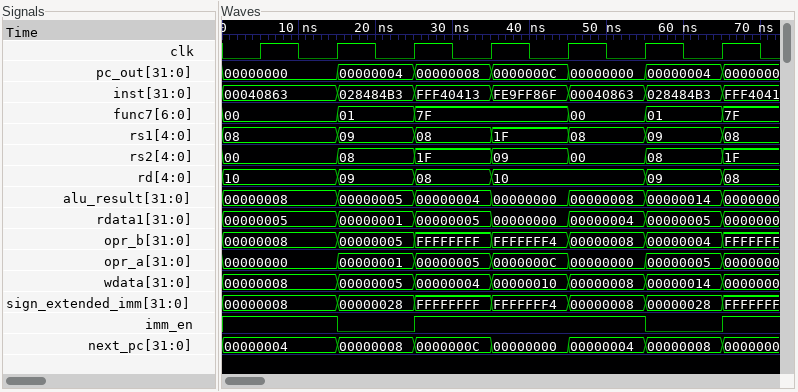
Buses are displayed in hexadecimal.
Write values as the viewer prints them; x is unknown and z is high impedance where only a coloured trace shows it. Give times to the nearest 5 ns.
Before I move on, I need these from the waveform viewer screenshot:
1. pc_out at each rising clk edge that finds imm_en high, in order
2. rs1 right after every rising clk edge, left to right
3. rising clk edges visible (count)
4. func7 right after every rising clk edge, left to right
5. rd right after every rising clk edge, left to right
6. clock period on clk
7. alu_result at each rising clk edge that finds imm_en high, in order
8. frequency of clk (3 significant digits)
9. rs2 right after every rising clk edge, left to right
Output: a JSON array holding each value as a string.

["00000000, 00000000, 00000008, 0000000C, 00000000", "08, 09, 08, 1F, 08, 09, 08", "7", "00, 01, 7F, 7F, 00, 01, 7F", "10, 09, 08, 10, 10, 09, 08", "10 ns", "00000008, 00000008, 00000004, 00000000, 00000008", "100 MHz", "00, 08, 1F, 09, 00, 08, 1F"]
